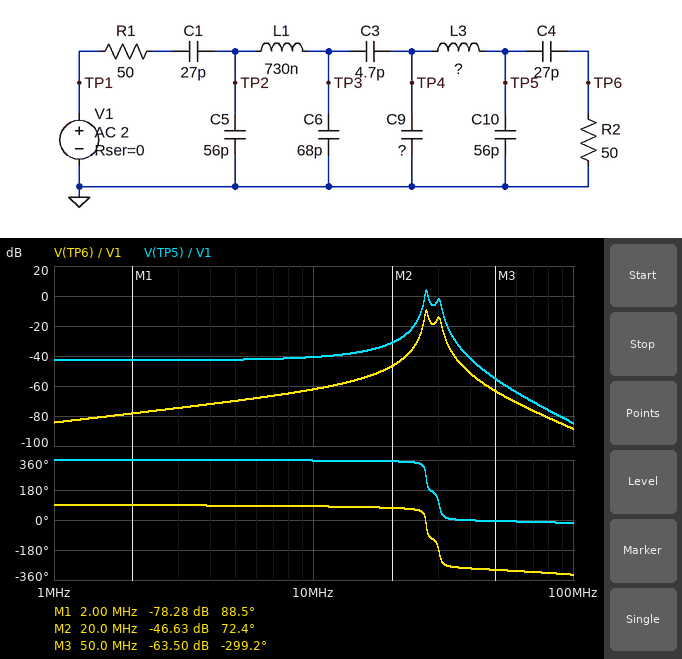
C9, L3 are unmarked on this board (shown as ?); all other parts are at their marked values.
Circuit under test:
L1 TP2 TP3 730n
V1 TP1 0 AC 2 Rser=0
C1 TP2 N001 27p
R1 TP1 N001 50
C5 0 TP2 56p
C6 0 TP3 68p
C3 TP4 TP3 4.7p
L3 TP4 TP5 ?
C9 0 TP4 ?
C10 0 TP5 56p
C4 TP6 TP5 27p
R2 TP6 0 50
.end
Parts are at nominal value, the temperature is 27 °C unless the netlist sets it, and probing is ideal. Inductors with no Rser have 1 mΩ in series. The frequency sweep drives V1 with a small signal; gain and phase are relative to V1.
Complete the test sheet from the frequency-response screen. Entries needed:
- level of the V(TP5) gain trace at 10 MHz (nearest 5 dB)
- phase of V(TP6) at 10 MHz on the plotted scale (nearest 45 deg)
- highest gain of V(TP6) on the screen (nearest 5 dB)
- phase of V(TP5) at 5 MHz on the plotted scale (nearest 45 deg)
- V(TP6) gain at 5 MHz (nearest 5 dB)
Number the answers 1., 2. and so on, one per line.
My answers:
1. -40 dB
2. 90 deg
3. -10 dB
4. 360 deg
5. -70 dB
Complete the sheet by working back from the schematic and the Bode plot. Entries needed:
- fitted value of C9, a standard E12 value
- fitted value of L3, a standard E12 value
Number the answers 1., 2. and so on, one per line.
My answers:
1. 27 pF
2. 1.5 µH
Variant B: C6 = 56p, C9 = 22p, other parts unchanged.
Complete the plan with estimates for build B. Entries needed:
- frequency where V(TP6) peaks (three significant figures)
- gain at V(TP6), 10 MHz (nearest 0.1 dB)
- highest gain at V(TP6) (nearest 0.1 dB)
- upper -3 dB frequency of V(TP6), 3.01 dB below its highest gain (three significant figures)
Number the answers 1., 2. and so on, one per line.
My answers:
1. 28.7 MHz
2. -61.3 dB
3. -7.5 dB
4. 29.0 MHz
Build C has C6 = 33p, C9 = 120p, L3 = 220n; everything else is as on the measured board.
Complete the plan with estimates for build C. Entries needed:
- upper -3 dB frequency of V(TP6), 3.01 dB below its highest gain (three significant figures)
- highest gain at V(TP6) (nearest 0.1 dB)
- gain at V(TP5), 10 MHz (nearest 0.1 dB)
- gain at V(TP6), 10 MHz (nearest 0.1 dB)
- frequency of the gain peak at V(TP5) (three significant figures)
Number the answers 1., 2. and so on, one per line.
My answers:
1. 37.3 MHz
2. -18.9 dB
3. -44.9 dB
4. -66.3 dB
5. 36.7 MHz
